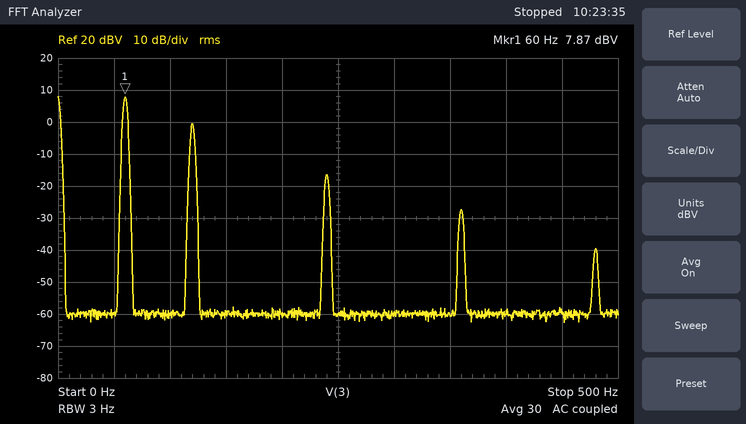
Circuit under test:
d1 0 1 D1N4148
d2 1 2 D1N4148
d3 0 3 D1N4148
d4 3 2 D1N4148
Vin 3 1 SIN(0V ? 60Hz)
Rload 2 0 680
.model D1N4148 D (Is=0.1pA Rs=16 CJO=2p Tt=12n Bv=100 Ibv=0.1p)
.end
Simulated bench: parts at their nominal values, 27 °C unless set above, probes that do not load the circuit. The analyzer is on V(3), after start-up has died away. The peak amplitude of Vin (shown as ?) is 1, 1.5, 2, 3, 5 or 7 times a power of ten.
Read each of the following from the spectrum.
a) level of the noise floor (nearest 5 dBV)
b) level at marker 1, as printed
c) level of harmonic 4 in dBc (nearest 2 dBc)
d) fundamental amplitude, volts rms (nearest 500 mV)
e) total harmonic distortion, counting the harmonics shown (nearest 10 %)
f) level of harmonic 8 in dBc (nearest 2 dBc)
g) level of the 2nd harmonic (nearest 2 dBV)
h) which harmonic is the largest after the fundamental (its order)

-60 dBV
7.87 dBV
-24 dBc
2.5 V
40 %
-48 dBc
0 dBV
2
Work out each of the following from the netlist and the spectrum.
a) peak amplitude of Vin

7 V
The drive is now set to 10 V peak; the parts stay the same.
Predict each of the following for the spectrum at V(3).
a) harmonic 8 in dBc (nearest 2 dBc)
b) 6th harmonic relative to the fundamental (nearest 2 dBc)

-40 dBc
-32 dBc
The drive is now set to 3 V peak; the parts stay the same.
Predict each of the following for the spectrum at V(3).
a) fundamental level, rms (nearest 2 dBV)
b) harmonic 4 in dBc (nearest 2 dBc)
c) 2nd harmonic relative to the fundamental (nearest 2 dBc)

0 dBV
-44 dBc
-10 dBc
